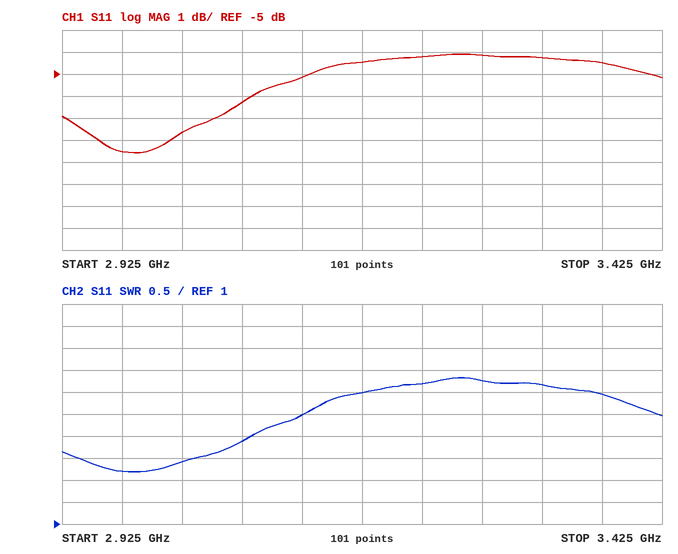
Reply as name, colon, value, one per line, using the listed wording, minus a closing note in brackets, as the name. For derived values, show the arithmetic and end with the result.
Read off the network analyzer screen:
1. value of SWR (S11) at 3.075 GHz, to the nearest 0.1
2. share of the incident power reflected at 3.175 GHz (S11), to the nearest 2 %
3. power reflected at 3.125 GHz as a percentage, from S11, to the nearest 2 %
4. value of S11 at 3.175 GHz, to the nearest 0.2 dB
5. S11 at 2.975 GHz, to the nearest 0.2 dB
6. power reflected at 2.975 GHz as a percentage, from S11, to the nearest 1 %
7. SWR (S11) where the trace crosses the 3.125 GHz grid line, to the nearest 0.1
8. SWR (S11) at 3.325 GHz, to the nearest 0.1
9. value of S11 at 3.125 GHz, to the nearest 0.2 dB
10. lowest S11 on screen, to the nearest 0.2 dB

value of SWR (S11) at 3.075 GHz, to the nearest 0.1: 2.9
share of the incident power reflected at 3.175 GHz (S11), to the nearest 2 %: 10^(-4.4/10) ≈ 36 %
power reflected at 3.125 GHz as a percentage, from S11, to the nearest 2 %: 10^(-5.2/10) ≈ 30 %
value of S11 at 3.175 GHz, to the nearest 0.2 dB: -4.4 dB
S11 at 2.975 GHz, to the nearest 0.2 dB: -8.6 dB
power reflected at 2.975 GHz as a percentage, from S11, to the nearest 1 %: 10^(-8.6/10) ≈ 14 %
SWR (S11) where the trace crosses the 3.125 GHz grid line, to the nearest 0.1: 3.5
SWR (S11) at 3.325 GHz, to the nearest 0.1: 4.2
value of S11 at 3.125 GHz, to the nearest 0.2 dB: -5.2 dB
lowest S11 on screen, to the nearest 0.2 dB: -8.6 dB
